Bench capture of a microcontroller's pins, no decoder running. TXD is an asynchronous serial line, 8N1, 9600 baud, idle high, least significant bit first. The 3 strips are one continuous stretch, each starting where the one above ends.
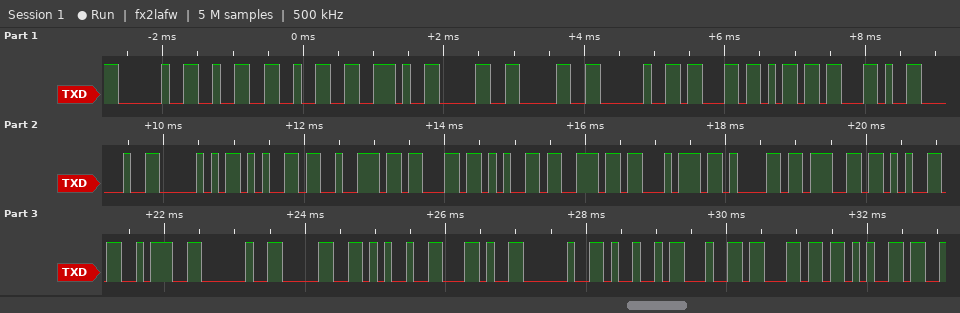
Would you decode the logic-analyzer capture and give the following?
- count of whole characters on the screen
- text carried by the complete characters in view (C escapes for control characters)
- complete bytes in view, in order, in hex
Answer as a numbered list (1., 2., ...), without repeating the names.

1. 31
2. " 22.00 cm, Percentage: 0%, Idle"
3. 0x20 0x32 0x32 0x2E 0x30 0x30 0x20 0x63 0x6D 0x2C 0x20 0x50 0x65 0x72 0x63 0x65 0x6E 0x74 0x61 0x67 0x65 0x3A 0x20 0x30 0x25 0x2C 0x20 0x49 0x64 0x6C 0x65
